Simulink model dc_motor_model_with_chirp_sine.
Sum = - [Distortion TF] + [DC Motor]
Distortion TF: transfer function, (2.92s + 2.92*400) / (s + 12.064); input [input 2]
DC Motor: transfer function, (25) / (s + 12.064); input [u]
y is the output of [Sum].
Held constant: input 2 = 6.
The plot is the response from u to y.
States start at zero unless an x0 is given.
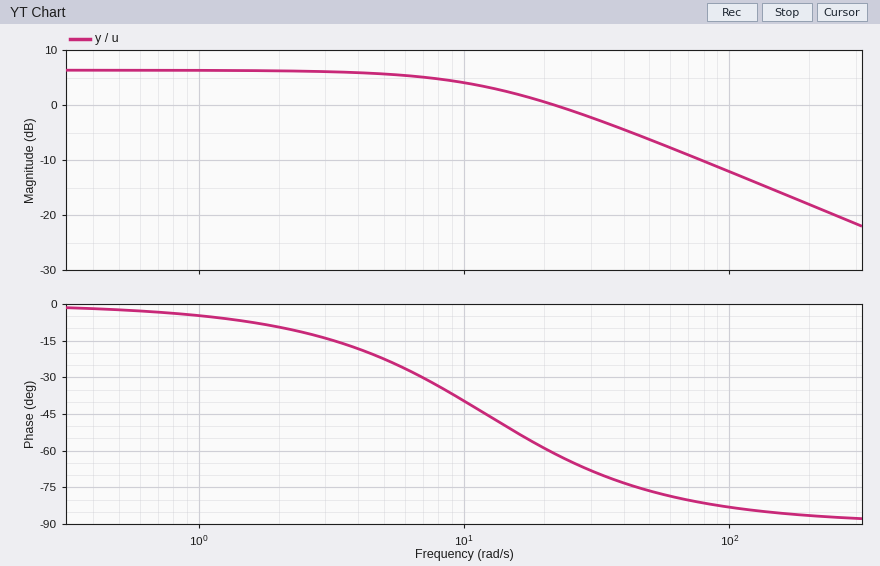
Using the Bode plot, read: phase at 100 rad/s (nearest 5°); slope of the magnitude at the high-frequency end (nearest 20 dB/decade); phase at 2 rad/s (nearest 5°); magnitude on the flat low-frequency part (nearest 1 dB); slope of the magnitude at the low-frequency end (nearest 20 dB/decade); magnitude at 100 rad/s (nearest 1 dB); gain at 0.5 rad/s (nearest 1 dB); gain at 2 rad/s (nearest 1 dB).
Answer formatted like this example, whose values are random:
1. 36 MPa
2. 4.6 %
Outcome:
1. -85°
2. -20 dB/decade
3. -10°
4. 6 dB
5. 0 dB/decade
6. -12 dB
7. 6 dB
8. 6 dB
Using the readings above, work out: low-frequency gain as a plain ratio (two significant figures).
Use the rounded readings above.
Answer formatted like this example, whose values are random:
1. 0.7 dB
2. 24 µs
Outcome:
1. 2.0
